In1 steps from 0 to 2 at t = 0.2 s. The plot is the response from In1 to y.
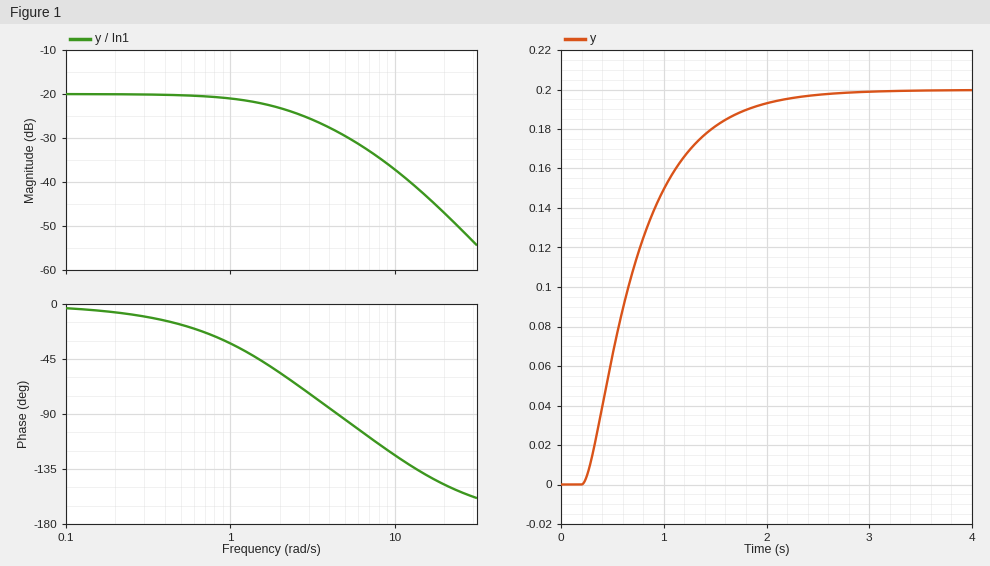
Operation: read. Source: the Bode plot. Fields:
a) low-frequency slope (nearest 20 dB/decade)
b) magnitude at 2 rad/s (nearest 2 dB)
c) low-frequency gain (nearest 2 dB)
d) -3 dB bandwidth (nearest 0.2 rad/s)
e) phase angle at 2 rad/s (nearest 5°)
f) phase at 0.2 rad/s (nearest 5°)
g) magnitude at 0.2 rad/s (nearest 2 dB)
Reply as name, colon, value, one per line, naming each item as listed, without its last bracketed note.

low-frequency slope: 0 dB/decade
magnitude at 2 rad/s: -24 dB
low-frequency gain: -20 dB
-3 dB bandwidth: 2.0 rad/s
phase angle at 2 rad/s: -55°
phase at 0.2 rad/s: -5°
magnitude at 0.2 rad/s: -20 dB
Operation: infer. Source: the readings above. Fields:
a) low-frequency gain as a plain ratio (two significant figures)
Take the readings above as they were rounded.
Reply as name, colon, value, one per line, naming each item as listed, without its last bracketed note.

low-frequency gain as a plain ratio: 0.10
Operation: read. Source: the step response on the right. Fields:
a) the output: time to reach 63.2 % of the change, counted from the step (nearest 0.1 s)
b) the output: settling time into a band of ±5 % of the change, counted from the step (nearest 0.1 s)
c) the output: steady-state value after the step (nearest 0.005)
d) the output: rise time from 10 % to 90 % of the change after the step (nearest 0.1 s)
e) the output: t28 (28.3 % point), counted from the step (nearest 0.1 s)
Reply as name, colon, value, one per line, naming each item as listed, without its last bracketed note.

the output: time to reach 63.2 % of the change, counted from the step: 0.6 s
the output: settling time into a band of ±5 % of the change, counted from the step: 1.6 s
the output: steady-state value after the step: 0.200
the output: rise time from 10 % to 90 % of the change after the step: 1.1 s
the output: t28 (28.3 % point), counted from the step: 0.3 s
